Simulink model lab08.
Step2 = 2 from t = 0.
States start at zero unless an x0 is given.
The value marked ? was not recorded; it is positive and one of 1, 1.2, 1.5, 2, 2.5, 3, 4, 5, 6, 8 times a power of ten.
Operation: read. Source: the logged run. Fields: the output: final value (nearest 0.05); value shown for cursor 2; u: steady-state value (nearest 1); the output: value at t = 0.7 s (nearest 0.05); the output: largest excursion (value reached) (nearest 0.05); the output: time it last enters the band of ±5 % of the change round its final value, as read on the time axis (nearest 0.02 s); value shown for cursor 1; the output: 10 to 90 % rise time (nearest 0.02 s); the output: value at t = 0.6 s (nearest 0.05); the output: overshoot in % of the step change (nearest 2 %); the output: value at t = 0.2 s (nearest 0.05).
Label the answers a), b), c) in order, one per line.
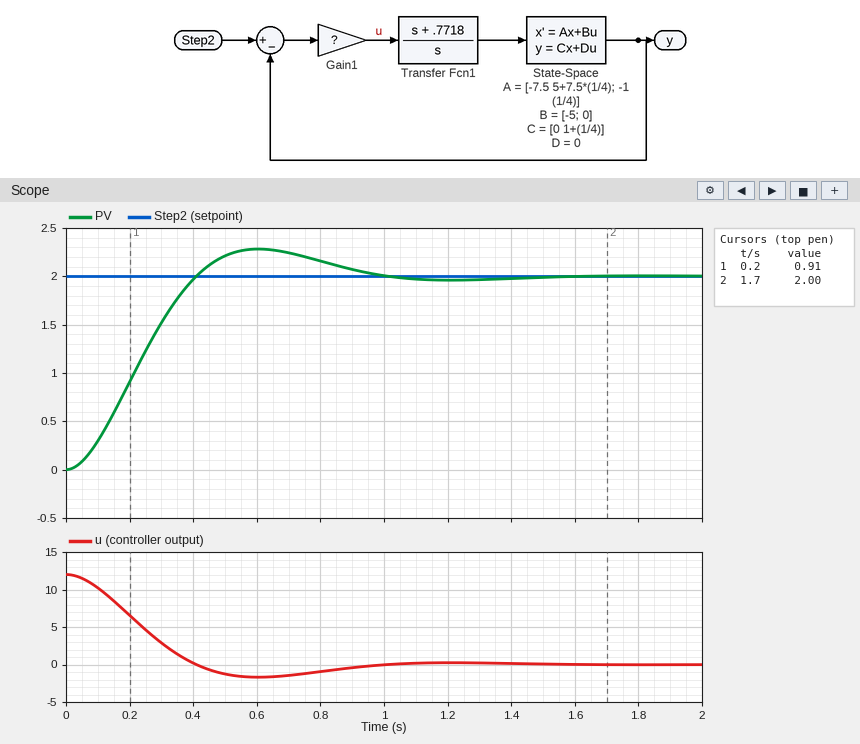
a) 2.00
b) 2.00
c) 0
d) 2.25
e) 2.30
f) 0.86 s
g) 0.91
h) 0.28 s
i) 2.30
j) 14 %
k) 0.90
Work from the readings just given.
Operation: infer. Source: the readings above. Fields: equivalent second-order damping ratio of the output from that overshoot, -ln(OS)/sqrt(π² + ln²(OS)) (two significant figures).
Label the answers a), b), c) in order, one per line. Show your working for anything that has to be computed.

a) ln(0.14) = -1.966; 1.966 / sqrt(9.870 + 3.866) = 0.53
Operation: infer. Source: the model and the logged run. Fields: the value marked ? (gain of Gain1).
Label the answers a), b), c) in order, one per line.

a) 6
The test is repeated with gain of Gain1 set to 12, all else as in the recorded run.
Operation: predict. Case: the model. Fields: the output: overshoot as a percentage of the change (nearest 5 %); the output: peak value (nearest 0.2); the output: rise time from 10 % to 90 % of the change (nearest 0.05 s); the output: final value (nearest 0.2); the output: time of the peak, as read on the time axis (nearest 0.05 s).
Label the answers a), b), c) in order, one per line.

a) 30 %
b) 2.6
c) 0.15 s
d) 2.0
e) 0.40 s
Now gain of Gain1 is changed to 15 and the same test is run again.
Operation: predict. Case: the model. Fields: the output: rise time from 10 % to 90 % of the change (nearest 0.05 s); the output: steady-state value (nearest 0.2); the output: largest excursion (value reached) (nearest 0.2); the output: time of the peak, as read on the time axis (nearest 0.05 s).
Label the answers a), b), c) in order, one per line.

a) 0.15 s
b) 2.0
c) 2.6
d) 0.35 s
